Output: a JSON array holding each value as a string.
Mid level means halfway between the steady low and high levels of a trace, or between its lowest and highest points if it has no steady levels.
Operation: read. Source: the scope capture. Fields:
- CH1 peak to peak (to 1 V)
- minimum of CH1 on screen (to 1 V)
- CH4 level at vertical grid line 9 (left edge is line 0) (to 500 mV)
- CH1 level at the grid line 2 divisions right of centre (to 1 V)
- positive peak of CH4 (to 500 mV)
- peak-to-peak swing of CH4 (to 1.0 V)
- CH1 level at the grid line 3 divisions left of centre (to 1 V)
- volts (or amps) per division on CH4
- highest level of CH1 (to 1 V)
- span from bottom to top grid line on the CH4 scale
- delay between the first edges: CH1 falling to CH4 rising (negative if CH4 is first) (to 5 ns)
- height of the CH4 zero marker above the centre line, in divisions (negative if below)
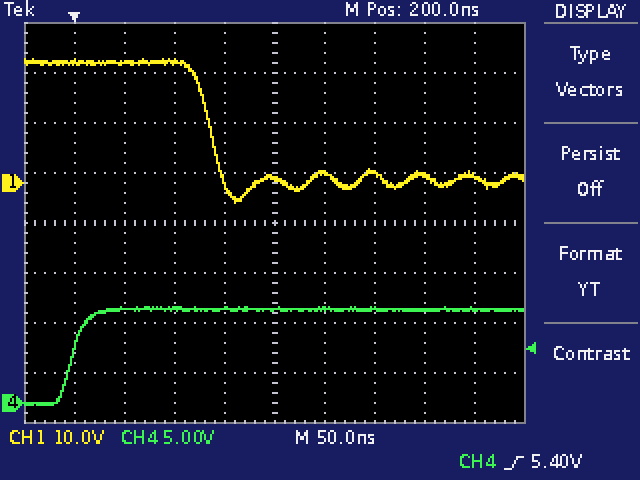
["29 V", "-4 V", "9.5 V", "2 V", "9.5 V", "10.0 V", "24 V", "5 V", "25 V", "40 V", "-140 ns", "-3.6 div"]
